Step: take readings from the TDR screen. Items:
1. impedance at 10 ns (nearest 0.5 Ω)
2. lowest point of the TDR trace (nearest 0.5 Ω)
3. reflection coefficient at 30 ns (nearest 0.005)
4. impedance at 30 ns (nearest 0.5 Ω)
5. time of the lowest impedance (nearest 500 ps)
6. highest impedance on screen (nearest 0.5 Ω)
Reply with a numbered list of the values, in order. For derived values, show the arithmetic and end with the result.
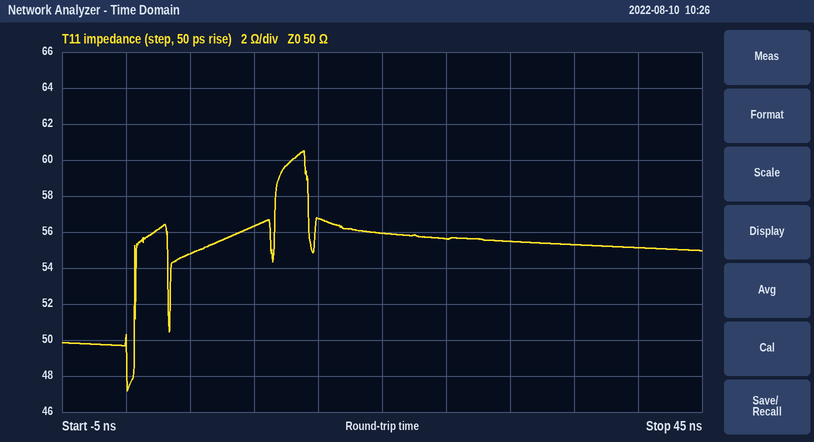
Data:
1. 56.5 Ω
2. 47.0 Ω
3. (55.5 − 50)/(55.5 + 50) ≈ +0.0521, so +0.050 to the nearest 0.005
4. 55.5 Ω
5. 0.0 ns
6. 60.5 Ω
